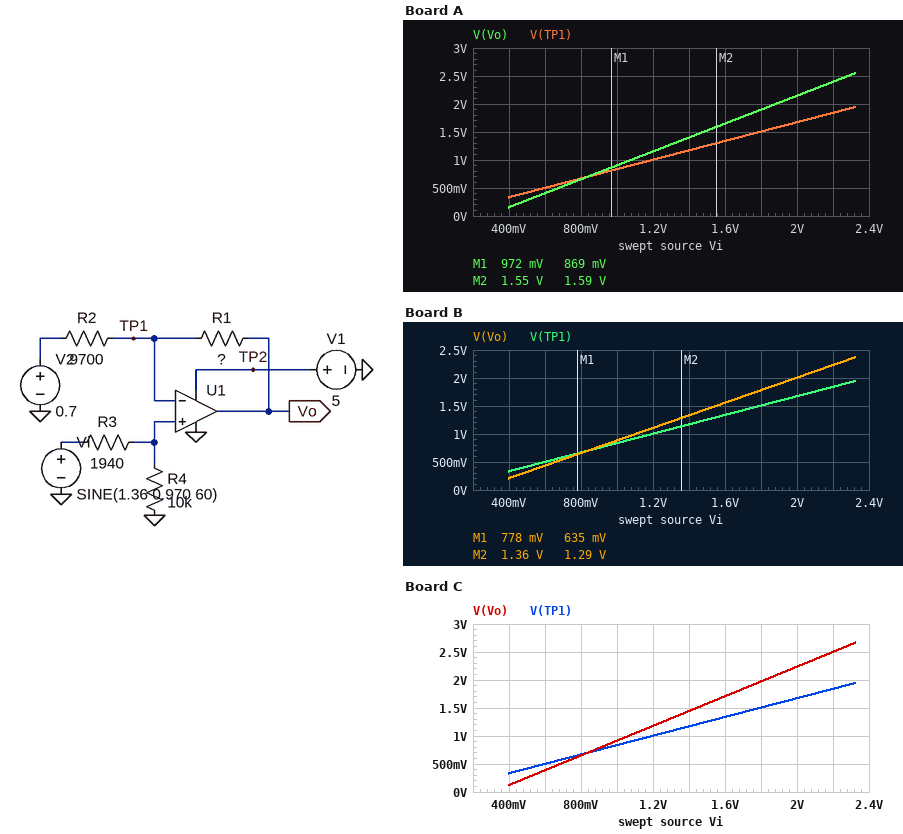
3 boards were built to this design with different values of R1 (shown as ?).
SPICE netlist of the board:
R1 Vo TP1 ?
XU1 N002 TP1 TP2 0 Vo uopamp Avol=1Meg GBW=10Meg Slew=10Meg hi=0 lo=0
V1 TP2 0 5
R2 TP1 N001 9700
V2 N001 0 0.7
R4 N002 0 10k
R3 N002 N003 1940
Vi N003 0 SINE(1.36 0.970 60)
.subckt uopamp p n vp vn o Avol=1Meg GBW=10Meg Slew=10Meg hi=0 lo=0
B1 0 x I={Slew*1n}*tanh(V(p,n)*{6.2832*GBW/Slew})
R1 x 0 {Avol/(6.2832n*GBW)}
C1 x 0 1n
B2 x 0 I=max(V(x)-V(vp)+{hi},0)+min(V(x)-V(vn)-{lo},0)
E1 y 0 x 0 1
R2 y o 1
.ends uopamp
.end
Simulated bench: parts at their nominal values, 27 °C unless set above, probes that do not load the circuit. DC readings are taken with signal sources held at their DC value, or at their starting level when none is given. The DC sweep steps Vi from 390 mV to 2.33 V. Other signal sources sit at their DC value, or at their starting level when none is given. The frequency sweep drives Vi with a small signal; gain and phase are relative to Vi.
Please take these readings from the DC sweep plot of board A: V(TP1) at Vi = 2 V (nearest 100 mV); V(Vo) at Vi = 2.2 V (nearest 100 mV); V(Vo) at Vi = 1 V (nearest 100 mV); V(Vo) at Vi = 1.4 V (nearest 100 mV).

1.7 V
2.4 V
900 mV
1.4 V
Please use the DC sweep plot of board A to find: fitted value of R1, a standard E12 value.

4.7 kΩ
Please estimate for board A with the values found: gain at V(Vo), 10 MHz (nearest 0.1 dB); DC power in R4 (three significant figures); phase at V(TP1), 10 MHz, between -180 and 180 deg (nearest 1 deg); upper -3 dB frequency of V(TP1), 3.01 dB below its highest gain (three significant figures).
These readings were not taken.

-3.2 dB
130 µW
-56 deg
6.74 MHz
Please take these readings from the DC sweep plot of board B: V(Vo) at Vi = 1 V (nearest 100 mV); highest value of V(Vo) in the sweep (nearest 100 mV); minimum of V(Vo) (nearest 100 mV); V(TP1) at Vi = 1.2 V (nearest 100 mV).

900 mV
2.4 V
200 mV
1.0 V
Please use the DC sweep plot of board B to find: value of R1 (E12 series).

3.3 kΩ
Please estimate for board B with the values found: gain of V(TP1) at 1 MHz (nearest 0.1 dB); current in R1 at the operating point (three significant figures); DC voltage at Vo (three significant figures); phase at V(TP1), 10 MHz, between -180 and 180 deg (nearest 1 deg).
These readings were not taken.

-1.6 dB
45.3 µA
1.29 V
-53 deg
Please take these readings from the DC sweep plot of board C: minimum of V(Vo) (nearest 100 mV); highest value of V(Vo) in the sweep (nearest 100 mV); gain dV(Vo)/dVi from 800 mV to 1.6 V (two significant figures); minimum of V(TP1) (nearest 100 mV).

100 mV
2.7 V
1.3 V/V
300 mV
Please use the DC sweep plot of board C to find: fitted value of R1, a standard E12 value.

5.6 kΩ
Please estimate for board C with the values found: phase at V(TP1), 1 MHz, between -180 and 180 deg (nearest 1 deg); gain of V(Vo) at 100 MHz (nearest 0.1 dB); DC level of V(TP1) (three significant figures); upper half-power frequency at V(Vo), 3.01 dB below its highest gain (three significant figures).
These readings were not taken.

-9 deg
-21.6 dB
1.14 V
6.34 MHz
